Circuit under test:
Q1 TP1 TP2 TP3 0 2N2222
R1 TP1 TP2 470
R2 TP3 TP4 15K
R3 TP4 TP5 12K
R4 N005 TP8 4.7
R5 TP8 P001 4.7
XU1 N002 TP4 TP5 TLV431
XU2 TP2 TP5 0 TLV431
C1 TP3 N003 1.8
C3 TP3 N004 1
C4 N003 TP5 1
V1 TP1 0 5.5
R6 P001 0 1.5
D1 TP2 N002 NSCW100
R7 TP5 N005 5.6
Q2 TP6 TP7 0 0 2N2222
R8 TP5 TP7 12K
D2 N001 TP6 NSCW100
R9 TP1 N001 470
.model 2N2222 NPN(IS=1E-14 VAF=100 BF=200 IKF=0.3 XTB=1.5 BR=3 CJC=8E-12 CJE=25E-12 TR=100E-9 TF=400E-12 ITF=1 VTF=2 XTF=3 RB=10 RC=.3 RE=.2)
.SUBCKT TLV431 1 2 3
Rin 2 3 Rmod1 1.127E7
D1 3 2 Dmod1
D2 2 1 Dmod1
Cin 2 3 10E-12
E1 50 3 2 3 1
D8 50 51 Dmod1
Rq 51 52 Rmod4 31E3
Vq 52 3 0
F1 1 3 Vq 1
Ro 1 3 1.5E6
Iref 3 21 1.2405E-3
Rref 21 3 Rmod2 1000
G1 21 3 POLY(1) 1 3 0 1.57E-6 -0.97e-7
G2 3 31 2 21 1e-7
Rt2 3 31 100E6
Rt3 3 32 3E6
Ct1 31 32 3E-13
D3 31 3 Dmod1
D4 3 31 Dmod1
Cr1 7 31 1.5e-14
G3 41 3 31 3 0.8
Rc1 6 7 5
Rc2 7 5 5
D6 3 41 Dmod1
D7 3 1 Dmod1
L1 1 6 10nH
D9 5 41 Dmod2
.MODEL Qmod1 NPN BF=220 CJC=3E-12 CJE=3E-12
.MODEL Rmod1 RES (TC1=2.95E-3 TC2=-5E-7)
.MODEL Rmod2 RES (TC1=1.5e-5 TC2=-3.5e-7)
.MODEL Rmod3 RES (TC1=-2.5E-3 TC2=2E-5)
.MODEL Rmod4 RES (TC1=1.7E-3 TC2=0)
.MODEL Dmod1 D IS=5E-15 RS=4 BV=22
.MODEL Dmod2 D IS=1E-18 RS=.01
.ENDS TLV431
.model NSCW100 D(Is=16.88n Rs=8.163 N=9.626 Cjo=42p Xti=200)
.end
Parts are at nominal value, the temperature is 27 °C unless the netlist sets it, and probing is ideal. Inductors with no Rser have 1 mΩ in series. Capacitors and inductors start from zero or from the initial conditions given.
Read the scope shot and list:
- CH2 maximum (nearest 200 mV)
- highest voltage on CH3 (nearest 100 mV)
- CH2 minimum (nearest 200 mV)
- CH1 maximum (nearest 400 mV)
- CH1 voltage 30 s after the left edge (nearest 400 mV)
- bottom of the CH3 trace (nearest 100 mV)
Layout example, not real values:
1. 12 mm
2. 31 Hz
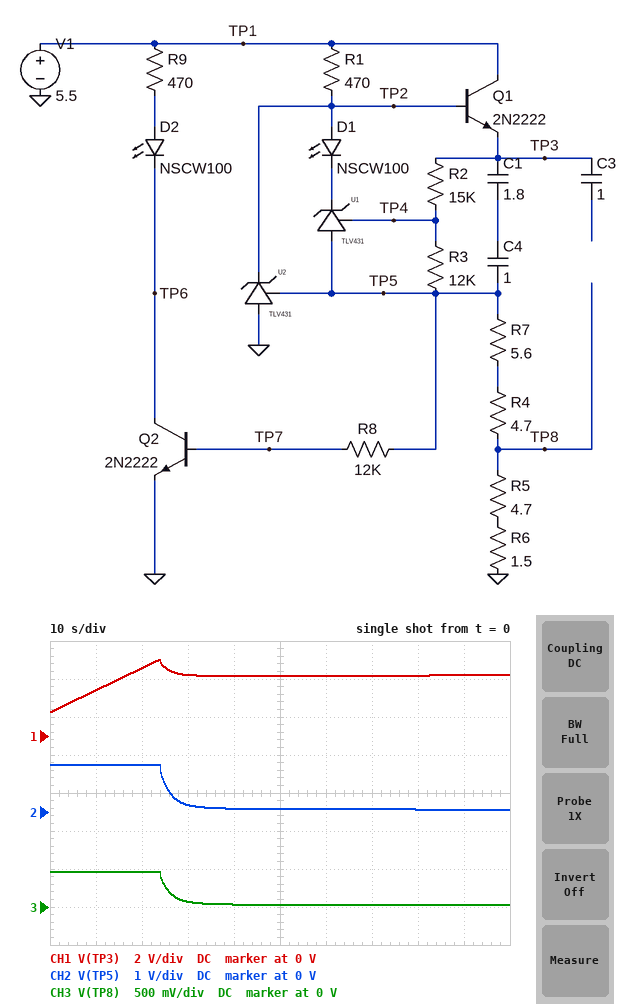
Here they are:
1. 1.2 V
2. 500 mV
3. 0 V
4. 4.0 V
5. 3.2 V
6. 0 V
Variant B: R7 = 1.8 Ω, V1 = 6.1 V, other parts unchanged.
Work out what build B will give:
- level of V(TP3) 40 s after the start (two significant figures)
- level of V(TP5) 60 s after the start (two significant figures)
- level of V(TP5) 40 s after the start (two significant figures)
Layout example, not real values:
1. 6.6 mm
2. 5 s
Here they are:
1. 3.2 V
2. 66 mV
3. 73 mV
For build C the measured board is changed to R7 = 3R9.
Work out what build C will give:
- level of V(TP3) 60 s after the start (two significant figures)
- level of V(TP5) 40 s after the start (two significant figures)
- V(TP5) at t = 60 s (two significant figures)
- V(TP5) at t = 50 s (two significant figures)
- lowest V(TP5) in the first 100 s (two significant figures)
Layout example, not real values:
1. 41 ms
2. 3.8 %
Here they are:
1. 3.2 V
2. 73 mV
3. 62 mV
4. 65 mV
5. 58 mV
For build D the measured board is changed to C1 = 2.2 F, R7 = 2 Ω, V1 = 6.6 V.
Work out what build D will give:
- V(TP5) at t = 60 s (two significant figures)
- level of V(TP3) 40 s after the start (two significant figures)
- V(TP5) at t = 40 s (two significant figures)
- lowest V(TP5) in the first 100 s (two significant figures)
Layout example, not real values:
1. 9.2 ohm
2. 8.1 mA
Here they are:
1. 80 mV
2. 3.3 V
3. 89 mV
4. 77 mV
